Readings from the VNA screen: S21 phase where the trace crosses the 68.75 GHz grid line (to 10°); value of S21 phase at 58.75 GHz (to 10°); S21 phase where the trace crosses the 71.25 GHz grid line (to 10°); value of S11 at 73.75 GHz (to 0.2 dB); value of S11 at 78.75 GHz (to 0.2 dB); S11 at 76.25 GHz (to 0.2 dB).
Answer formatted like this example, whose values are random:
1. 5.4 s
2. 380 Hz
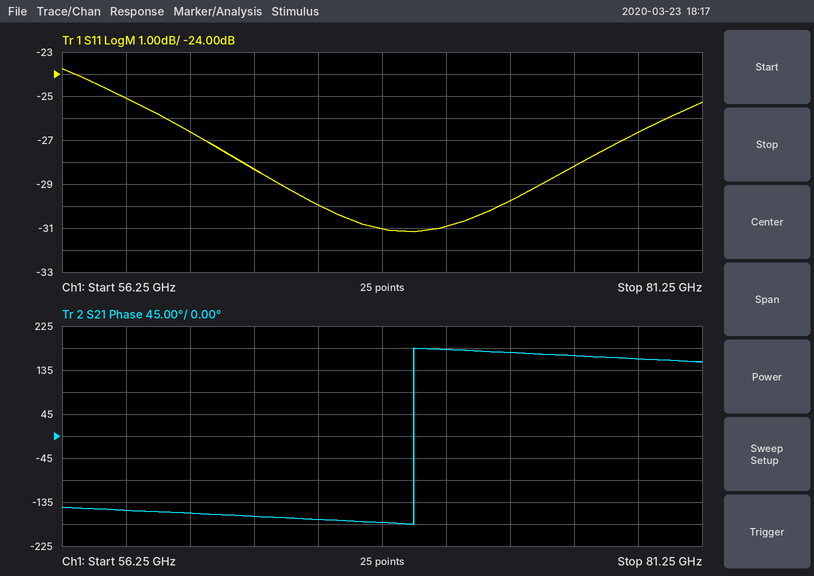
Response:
1. -180°
2. -150°
3. 180°
4. -29.8 dB
5. -26.6 dB
6. -28.2 dB
